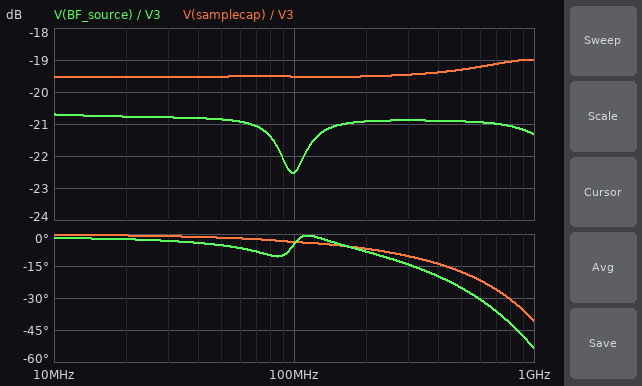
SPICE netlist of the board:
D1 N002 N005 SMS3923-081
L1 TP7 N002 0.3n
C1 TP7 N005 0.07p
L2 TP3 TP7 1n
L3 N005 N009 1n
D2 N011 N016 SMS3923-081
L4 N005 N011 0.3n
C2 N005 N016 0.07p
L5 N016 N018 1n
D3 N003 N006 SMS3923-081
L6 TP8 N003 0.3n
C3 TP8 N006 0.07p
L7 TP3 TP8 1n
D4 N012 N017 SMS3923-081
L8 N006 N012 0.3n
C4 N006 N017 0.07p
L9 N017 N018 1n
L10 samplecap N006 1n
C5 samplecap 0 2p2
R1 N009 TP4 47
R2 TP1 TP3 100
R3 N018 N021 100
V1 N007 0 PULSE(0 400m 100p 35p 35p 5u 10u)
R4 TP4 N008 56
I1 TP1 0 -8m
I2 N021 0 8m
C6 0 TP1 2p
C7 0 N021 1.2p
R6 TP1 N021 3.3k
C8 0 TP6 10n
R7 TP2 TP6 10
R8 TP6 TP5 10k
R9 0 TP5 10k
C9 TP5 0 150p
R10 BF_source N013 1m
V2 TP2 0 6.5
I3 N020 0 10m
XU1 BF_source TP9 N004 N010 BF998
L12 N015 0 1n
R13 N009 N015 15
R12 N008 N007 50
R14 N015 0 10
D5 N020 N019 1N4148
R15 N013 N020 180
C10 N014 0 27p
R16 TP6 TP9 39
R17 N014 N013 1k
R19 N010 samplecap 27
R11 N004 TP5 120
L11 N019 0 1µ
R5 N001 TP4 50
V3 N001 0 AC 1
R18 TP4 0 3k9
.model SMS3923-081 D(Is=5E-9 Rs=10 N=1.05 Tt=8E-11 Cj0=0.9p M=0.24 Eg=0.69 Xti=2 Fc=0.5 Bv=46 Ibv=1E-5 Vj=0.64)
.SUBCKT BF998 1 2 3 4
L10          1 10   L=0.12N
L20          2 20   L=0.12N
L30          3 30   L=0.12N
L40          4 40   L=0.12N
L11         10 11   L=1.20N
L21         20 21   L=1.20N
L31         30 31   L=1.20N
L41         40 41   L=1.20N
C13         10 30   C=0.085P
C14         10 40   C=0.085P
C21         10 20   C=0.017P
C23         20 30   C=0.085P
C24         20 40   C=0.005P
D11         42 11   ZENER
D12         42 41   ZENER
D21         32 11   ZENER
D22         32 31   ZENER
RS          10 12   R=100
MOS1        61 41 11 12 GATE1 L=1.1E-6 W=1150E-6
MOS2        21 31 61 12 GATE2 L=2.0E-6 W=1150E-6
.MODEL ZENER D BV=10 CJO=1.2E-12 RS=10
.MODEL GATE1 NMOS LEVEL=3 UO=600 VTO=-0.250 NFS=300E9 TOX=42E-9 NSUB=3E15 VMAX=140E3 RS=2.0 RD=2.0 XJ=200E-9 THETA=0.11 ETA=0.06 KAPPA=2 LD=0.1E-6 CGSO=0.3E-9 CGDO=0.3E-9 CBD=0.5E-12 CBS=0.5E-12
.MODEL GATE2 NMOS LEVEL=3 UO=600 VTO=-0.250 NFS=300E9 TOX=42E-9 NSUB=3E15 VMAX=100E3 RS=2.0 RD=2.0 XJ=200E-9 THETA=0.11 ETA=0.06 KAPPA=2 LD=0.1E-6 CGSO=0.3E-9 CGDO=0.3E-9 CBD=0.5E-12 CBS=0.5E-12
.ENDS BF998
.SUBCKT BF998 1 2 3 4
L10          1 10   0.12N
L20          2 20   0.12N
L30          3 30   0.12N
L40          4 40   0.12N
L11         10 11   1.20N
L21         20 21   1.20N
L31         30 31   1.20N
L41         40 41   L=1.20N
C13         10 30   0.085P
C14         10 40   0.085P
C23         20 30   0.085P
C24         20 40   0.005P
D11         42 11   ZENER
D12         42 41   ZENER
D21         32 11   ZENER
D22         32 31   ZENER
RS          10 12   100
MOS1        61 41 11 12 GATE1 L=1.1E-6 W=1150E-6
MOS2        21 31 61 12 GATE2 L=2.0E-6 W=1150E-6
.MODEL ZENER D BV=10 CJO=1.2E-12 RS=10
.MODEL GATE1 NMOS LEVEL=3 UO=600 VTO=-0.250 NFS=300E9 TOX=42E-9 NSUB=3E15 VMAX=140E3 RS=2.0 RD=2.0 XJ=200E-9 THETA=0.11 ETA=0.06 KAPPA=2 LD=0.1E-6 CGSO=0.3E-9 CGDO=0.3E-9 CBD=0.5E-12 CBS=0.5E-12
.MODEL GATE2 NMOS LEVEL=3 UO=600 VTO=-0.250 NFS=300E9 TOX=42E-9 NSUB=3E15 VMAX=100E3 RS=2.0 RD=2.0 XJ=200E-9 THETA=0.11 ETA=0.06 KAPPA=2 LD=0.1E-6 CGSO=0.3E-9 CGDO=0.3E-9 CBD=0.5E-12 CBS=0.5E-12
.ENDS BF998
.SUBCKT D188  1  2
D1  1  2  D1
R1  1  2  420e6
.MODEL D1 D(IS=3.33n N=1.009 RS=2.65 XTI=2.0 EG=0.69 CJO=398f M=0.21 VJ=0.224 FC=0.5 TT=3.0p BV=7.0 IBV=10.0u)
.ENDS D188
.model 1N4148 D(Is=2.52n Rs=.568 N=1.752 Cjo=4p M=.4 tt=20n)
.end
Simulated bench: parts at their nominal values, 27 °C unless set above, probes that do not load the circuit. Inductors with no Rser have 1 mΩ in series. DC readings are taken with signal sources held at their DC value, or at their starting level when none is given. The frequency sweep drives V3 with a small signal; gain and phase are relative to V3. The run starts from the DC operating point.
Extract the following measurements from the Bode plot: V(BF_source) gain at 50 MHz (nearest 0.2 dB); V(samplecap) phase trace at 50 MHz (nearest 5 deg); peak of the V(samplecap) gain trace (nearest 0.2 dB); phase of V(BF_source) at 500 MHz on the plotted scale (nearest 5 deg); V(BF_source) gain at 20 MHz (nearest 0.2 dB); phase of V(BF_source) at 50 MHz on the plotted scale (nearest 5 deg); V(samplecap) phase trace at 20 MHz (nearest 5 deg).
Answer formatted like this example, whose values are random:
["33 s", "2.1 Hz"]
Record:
["-20.8 dB", "0 deg", "-19.0 dB", "-25 deg", "-20.8 dB", "-5 deg", "0 deg"]
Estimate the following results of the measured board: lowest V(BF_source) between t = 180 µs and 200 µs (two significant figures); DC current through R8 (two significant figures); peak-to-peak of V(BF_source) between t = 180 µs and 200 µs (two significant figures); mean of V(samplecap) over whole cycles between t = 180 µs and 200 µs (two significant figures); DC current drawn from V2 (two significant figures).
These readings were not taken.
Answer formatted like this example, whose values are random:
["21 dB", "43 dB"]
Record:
["-110 mV", "320 µA", "18 mV", "10 mV", "10 mA"]
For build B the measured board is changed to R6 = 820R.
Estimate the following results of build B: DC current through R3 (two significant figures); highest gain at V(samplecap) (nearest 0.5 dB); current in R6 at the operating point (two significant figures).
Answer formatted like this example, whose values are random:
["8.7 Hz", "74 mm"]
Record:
["5.7 mA", "-19.5 dB", "2.3 mA"]
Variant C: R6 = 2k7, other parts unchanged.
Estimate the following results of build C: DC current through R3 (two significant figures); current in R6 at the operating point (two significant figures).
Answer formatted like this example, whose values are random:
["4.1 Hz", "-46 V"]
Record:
["7.2 mA", "830 µA"]
